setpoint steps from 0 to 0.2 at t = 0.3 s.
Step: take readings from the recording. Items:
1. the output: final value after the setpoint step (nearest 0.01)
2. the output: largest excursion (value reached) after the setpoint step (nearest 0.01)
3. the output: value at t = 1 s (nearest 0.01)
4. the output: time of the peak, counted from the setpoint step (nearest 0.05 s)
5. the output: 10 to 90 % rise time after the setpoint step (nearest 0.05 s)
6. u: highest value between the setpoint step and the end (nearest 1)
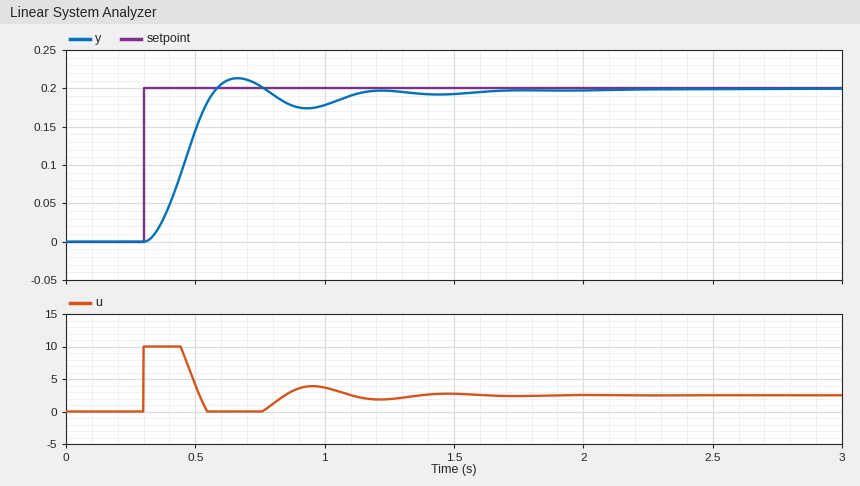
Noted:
0.20
0.21
0.18
0.35 s
0.20 s
10
